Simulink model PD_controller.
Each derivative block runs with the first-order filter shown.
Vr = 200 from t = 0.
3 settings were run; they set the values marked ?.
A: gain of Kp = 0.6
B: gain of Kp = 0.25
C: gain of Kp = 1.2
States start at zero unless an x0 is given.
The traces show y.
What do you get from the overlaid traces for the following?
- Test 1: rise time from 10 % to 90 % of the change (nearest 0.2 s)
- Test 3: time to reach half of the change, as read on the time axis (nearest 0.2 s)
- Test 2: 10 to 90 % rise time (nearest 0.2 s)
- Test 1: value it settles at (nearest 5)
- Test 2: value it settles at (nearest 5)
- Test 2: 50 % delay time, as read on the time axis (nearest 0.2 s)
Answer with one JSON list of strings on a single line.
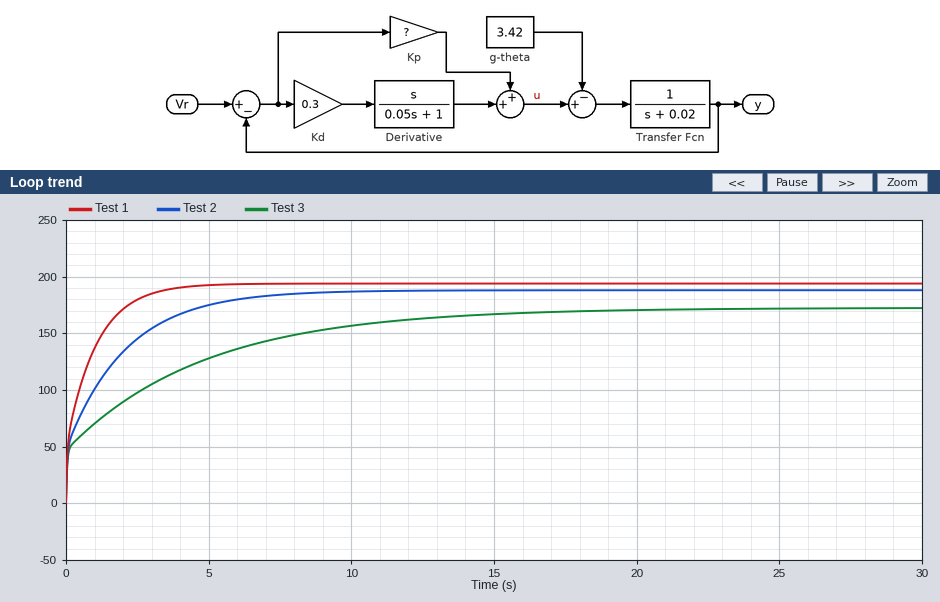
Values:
["2.2 s", "1.8 s", "4.2 s", "195", "190", "0.8 s"]
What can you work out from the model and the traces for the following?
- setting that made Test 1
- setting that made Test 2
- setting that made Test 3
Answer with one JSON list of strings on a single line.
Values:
["C", "A", "B"]
